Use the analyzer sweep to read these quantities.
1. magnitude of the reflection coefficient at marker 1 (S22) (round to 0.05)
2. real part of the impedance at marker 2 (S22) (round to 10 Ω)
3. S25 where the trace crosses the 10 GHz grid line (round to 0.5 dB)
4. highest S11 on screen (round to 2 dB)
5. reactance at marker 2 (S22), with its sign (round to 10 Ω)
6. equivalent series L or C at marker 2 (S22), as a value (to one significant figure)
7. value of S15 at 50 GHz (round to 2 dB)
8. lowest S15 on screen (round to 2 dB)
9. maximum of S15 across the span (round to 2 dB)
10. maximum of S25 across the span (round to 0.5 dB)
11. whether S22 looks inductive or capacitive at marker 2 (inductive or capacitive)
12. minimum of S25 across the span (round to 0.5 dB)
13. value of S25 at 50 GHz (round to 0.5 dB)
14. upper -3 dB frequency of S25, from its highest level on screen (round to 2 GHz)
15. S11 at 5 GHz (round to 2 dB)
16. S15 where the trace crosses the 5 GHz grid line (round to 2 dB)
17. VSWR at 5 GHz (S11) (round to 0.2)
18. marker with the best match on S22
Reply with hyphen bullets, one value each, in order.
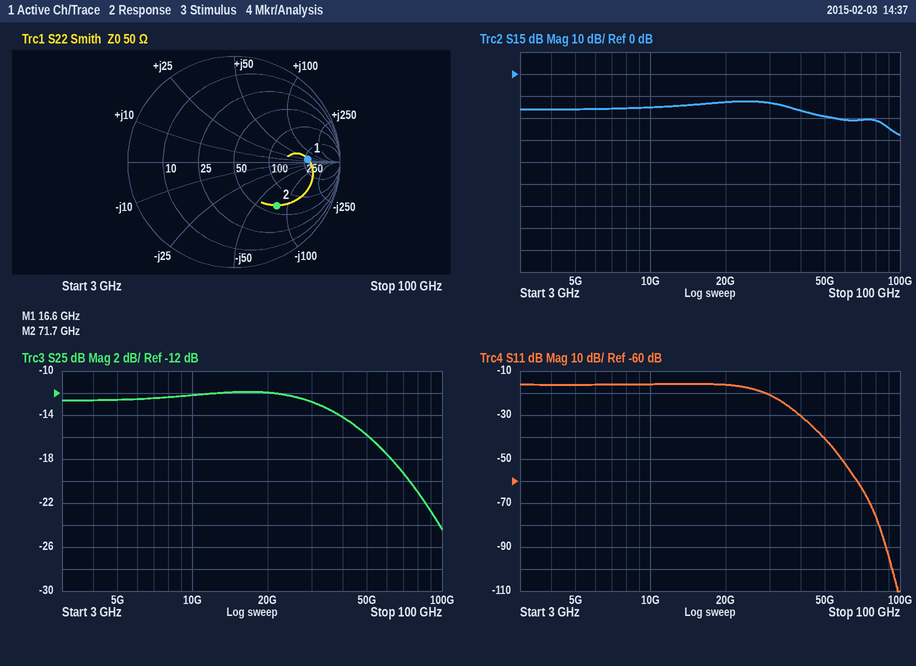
- 0.70
- 60 Ω
- -12.0 dB
- -16 dB
- -80 Ω
- 30 fF
- -20 dB
- -28 dB
- -12 dB
- -12.0 dB
- capacitive
- -24.5 dB
- -16.0 dB
- 44 GHz
- -16 dB
- -16 dB
- 1.4
- marker 2
